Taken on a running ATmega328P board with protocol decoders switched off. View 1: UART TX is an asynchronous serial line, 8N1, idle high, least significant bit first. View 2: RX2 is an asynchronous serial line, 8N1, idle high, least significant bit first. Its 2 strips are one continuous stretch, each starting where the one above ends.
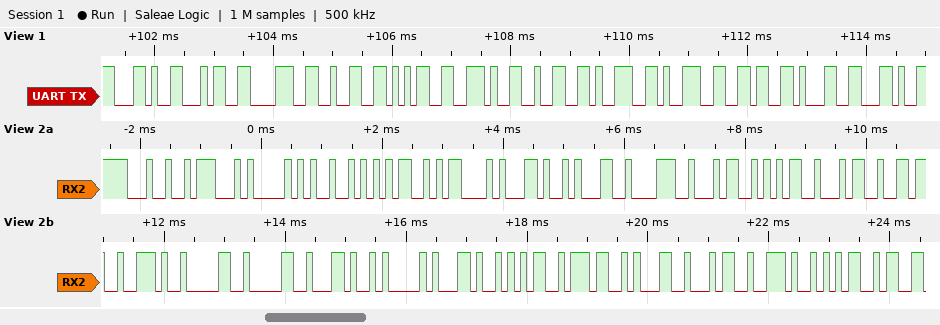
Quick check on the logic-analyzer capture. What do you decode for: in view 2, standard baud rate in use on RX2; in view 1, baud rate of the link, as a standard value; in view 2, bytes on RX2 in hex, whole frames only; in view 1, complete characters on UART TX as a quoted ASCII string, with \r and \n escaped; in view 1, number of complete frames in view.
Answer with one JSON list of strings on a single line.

["9600 baud", "9600 baud", "24 47 50 52 4D 43 2C 31 38 34 35 34 36 2E 30 30 2C 41 2C 35 37 31 34 2E 35", "\",4825.29961,\"", "12"]
